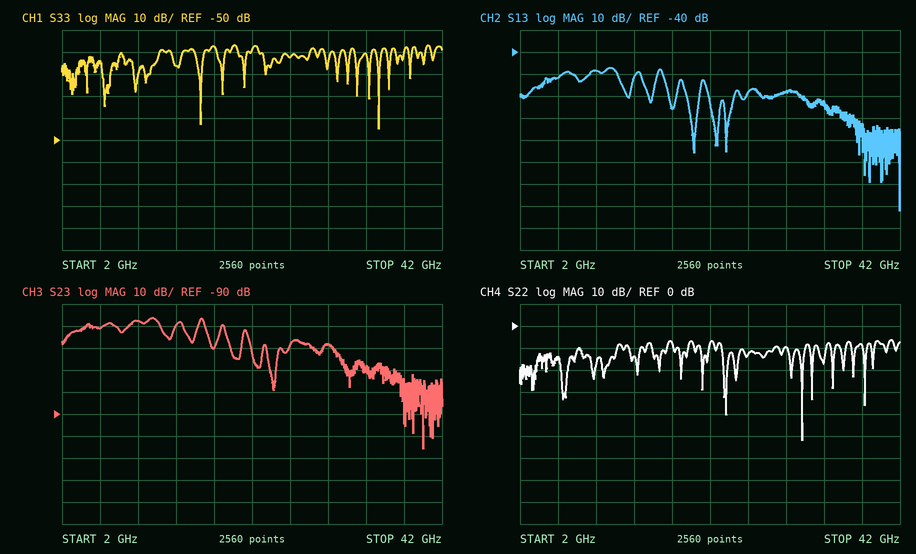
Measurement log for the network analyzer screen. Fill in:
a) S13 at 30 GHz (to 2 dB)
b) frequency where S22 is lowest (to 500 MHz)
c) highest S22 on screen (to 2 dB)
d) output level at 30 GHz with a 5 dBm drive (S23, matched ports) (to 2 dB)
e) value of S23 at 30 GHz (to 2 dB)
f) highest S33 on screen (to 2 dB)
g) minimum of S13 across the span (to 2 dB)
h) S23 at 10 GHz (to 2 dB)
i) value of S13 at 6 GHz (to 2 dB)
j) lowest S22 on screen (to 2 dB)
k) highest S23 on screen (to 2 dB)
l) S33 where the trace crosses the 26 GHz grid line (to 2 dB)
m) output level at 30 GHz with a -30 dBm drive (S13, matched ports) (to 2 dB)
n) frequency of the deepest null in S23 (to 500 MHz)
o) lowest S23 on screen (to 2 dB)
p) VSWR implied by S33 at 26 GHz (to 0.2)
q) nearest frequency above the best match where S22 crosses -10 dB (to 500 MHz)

-58 dB
31.5 GHz
-6 dB
-54 dBm
-58 dB
-6 dB
-112 dB
-48 dB
-52 dB
-52 dB
-46 dB
-12 dB
-88 dBm
40.0 GHz
-106 dB
1.6
32.0 GHz
